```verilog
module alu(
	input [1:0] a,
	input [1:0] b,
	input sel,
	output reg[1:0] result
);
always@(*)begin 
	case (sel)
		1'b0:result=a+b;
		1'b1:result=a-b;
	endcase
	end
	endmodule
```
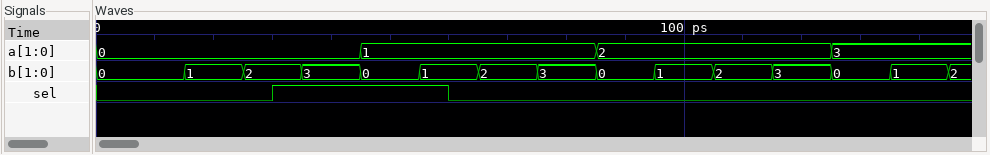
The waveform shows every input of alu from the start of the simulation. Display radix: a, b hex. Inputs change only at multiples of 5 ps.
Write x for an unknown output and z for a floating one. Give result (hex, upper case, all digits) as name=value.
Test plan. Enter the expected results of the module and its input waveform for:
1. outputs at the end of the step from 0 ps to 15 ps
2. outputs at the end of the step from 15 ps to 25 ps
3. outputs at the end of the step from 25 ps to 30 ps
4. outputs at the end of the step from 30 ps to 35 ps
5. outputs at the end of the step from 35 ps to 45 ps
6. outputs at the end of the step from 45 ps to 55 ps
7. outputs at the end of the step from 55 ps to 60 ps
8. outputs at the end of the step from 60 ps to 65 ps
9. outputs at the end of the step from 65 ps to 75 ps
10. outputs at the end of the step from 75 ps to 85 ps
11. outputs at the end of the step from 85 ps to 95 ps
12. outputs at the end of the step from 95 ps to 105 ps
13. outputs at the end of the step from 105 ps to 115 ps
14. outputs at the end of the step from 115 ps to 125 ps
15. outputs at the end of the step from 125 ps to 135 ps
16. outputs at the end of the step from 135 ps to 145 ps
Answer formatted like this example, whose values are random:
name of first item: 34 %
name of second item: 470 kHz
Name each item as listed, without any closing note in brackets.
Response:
outputs at the end of the step from 0 ps to 15 ps: result=0
outputs at the end of the step from 15 ps to 25 ps: result=1
outputs at the end of the step from 25 ps to 30 ps: result=2
outputs at the end of the step from 30 ps to 35 ps: result=2
outputs at the end of the step from 35 ps to 45 ps: result=1
outputs at the end of the step from 45 ps to 55 ps: result=1
outputs at the end of the step from 55 ps to 60 ps: result=0
outputs at the end of the step from 60 ps to 65 ps: result=2
outputs at the end of the step from 65 ps to 75 ps: result=3
outputs at the end of the step from 75 ps to 85 ps: result=0
outputs at the end of the step from 85 ps to 95 ps: result=2
outputs at the end of the step from 95 ps to 105 ps: result=3
outputs at the end of the step from 105 ps to 115 ps: result=0
outputs at the end of the step from 115 ps to 125 ps: result=1
outputs at the end of the step from 125 ps to 135 ps: result=3
outputs at the end of the step from 135 ps to 145 ps: result=0
